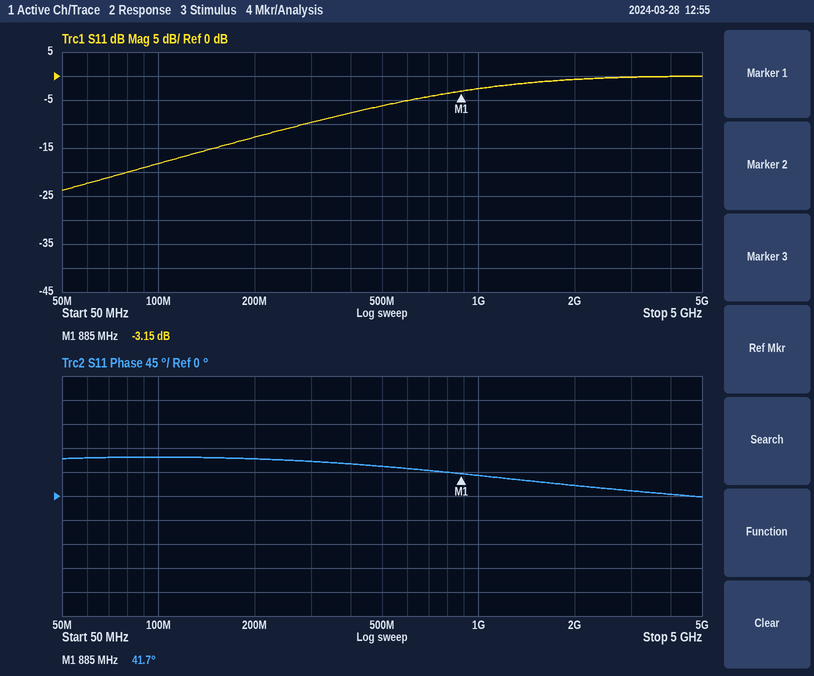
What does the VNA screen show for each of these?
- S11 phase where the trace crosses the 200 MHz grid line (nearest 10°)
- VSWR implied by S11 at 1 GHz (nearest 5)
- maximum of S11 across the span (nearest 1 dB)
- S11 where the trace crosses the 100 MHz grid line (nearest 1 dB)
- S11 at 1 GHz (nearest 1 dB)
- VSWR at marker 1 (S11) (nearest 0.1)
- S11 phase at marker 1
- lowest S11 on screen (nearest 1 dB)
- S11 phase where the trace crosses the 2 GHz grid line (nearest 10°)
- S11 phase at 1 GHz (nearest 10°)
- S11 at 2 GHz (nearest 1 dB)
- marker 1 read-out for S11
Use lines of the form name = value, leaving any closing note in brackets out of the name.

S11 phase where the trace crosses the 200 MHz grid line = 70°
VSWR implied by S11 at 1 GHz = 5
maximum of S11 across the span = 0 dB
S11 where the trace crosses the 100 MHz grid line = -18 dB
S11 at 1 GHz = -3 dB
VSWR at marker 1 (S11) = 5.6
S11 phase at marker 1 = 41.7°
lowest S11 on screen = -24 dB
S11 phase where the trace crosses the 2 GHz grid line = 20°
S11 phase at 1 GHz = 40°
S11 at 2 GHz = -1 dB
marker 1 read-out for S11 = -3.15 dB
